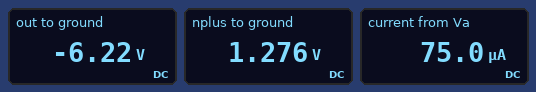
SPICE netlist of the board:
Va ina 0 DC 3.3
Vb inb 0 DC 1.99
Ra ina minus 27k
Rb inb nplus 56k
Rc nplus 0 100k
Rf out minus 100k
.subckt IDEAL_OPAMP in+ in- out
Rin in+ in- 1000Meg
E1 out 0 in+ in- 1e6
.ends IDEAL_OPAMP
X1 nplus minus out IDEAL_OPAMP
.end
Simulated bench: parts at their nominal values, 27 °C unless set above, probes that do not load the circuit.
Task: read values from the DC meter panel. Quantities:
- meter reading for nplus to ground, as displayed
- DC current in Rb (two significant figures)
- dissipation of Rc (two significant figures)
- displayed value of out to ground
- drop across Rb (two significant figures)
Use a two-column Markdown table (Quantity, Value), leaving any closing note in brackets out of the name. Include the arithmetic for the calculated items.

| Quantity | Value |
|---|---|
| meter reading for nplus to ground, as displayed | 1.276 V |
| DC current in Rb | (1.99 V - 1.276 V) / 56 kΩ = 13 µA |
| dissipation of Rc | (1.276 V)^2 / 100 kΩ = 16 µW |
| displayed value of out to ground | -6.22 V |
| drop across Rb | 1.99 V - 1.276 V = 710 mV |
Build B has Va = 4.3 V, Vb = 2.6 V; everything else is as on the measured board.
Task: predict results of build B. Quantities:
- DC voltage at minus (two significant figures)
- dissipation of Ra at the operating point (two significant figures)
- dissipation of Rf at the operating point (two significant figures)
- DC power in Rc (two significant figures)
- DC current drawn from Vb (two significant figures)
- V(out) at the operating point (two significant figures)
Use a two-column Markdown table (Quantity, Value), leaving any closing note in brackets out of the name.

| Quantity | Value |
|---|---|
| DC voltage at minus | 1.7 V |
| dissipation of Ra at the operating point | 260 µW |
| dissipation of Rf at the operating point | 950 µW |
| DC power in Rc | 28 µW |
| DC current drawn from Vb | 17 µA |
| V(out) at the operating point | -8.1 V |
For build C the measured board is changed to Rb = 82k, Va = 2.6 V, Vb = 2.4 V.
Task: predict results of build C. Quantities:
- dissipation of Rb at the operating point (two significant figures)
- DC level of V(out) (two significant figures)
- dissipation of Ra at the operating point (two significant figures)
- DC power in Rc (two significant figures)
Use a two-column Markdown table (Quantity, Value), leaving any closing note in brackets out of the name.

| Quantity | Value |
|---|---|
| dissipation of Rb at the operating point | 14 µW |
| DC level of V(out) | -3.4 V |
| dissipation of Ra at the operating point | 61 µW |
| DC power in Rc | 17 µW |
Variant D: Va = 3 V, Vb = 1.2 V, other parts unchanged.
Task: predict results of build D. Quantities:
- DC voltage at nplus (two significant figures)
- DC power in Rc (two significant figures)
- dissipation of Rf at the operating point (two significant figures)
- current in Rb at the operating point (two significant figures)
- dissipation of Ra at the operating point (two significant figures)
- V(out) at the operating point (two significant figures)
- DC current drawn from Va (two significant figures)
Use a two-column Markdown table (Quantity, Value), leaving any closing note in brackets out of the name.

| Quantity | Value |
|---|---|
| DC voltage at nplus | 770 mV |
| DC power in Rc | 5.9 µW |
| dissipation of Rf at the operating point | 680 µW |
| current in Rb at the operating point | 7.7 µA |
| dissipation of Ra at the operating point | 180 µW |
| V(out) at the operating point | -7.5 V |
| DC current drawn from Va | 83 µA |
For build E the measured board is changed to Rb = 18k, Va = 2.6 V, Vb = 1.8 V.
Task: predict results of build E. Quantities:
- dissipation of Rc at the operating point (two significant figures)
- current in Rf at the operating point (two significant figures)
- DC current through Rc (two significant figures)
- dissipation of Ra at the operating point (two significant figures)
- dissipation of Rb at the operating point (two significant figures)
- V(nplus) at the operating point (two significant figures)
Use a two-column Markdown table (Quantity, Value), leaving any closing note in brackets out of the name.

| Quantity | Value |
|---|---|
| dissipation of Rc at the operating point | 23 µW |
| current in Rf at the operating point | 40 µA |
| DC current through Rc | 15 µA |
| dissipation of Ra at the operating point | 43 µW |
| dissipation of Rb at the operating point | 4.2 µW |
| V(nplus) at the operating point | 1.5 V |
